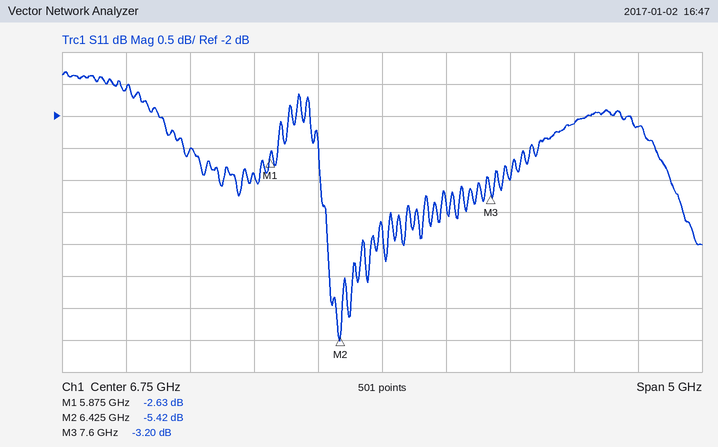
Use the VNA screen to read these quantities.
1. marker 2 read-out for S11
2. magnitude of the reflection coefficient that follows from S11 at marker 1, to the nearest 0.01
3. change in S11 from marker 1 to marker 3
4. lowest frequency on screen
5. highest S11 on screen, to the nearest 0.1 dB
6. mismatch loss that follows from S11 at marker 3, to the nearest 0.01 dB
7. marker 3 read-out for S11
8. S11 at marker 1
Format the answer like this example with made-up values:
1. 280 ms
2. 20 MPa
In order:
1. -5.42 dB
2. 0.74
3. -0.57 dB
4. 4.25 GHz
5. -1.3 dB
6. 2.83 dB
7. -3.20 dB
8. -2.63 dB
